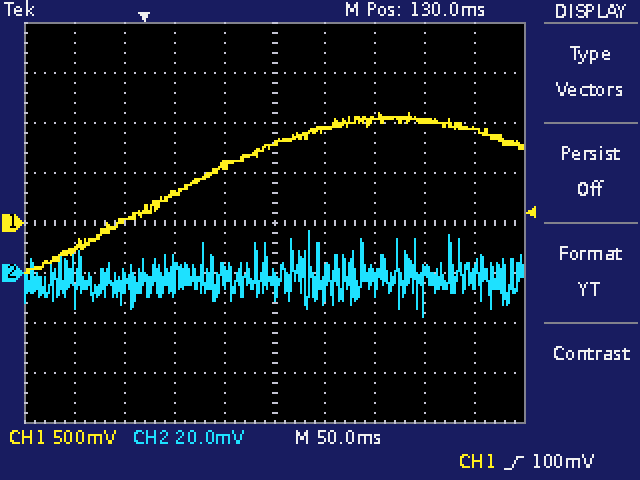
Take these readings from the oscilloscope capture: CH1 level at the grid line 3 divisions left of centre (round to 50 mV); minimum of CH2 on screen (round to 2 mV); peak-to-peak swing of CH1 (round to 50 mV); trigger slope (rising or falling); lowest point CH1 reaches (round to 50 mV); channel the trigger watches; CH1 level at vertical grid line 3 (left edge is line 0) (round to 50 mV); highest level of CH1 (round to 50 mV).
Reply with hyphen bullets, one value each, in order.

- 0 mV
- -18 mV
- 1.60 V
- rising
- -500 mV
- CH1
- 300 mV
- 1.10 V
